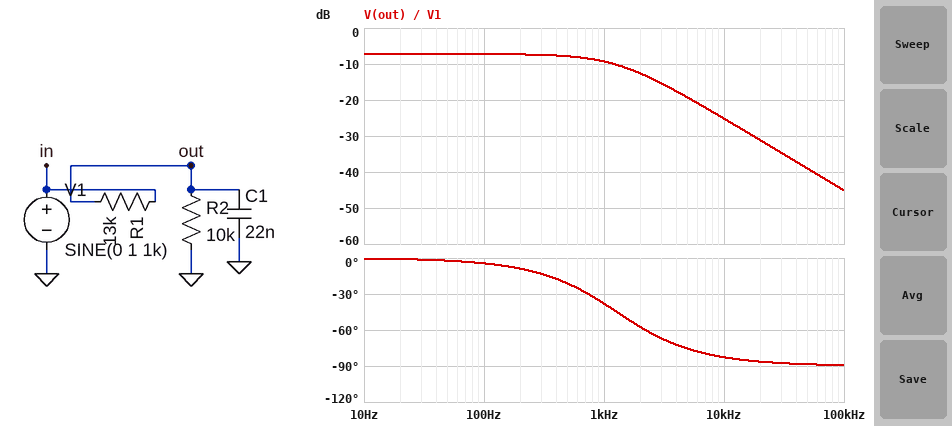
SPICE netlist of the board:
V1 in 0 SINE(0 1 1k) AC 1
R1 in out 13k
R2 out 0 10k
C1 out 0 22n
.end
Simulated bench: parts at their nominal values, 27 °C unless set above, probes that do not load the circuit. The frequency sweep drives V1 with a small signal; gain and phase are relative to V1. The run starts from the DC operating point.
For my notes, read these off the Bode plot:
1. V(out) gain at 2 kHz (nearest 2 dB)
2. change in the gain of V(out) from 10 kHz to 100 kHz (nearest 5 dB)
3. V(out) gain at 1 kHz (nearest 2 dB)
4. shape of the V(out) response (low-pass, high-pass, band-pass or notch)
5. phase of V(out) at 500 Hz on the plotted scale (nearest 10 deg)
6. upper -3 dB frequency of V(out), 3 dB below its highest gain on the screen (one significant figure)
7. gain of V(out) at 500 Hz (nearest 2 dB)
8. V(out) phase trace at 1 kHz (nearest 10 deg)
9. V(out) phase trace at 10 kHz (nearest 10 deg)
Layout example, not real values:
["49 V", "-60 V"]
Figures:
["-12 dB", "-20 dB", "-10 dB", "low-pass", "-20 deg", "1 kHz", "-8 dB", "-40 deg", "-80 deg"]
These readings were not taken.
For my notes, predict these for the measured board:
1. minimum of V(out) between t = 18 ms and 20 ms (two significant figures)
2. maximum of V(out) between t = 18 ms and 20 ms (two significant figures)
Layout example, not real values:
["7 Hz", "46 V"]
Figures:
["-340 mV", "340 mV"]
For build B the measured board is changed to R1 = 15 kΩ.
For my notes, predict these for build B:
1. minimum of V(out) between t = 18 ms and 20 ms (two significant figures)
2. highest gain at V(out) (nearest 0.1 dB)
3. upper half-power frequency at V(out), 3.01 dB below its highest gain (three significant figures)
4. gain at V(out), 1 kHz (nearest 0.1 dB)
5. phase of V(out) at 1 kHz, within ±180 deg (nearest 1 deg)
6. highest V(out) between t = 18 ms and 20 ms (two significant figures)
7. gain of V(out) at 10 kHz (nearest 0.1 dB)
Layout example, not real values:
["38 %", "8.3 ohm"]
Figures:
["-310 mV", "-8.0 dB", "1.21 kHz", "-10.2 dB", "-40 deg", "310 mV", "-26.4 dB"]
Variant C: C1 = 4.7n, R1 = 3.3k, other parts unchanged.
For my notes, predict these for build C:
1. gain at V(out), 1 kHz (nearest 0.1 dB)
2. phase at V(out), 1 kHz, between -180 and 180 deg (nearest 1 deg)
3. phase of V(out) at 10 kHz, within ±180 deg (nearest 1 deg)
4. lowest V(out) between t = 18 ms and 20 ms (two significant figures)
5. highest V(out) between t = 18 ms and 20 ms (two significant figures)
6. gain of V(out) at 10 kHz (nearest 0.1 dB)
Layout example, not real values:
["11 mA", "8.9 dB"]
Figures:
["-2.5 dB", "-4 deg", "-36 deg", "-750 mV", "750 mV", "-4.3 dB"]
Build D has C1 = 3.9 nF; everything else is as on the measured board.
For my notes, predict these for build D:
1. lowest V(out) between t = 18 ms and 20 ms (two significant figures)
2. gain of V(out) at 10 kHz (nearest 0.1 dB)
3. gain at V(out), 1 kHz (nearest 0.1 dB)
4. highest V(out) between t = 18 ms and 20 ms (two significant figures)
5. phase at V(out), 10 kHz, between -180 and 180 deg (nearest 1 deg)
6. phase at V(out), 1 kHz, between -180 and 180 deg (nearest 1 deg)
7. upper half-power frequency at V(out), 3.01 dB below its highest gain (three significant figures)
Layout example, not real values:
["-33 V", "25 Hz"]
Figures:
["-430 mV", "-11.9 dB", "-7.3 dB", "430 mV", "-54 deg", "-8 deg", "7.22 kHz"]
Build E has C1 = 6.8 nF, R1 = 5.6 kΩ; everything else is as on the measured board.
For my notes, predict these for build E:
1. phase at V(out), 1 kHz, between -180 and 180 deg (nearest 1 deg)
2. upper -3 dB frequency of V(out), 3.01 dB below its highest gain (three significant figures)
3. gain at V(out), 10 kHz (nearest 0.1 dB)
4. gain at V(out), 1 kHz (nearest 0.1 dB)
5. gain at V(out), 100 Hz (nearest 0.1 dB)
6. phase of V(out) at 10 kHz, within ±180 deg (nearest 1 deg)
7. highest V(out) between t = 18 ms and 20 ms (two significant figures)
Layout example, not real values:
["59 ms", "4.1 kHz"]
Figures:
["-9 deg", "6.52 kHz", "-9.1 dB", "-4.0 dB", "-3.9 dB", "-57 deg", "630 mV"]
